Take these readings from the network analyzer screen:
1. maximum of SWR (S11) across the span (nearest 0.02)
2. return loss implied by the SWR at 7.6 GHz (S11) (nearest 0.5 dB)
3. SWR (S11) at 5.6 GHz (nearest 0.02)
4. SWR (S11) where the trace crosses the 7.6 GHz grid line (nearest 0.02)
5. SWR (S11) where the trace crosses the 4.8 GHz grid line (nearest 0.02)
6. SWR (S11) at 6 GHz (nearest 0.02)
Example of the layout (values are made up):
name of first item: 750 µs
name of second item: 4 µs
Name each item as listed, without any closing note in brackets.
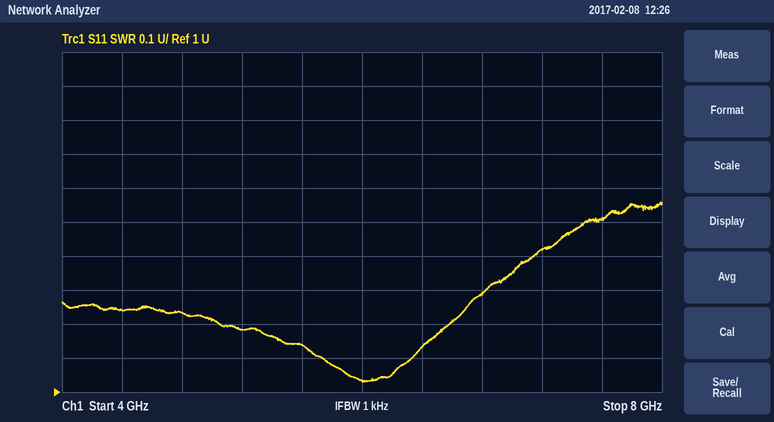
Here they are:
maximum of SWR (S11) across the span: 1.56
return loss implied by the SWR at 7.6 GHz (S11): 14.0 dB
SWR (S11) at 5.6 GHz: 1.14
SWR (S11) where the trace crosses the 7.6 GHz grid line: 1.50
SWR (S11) where the trace crosses the 4.8 GHz grid line: 1.24
SWR (S11) at 6 GHz: 1.04
